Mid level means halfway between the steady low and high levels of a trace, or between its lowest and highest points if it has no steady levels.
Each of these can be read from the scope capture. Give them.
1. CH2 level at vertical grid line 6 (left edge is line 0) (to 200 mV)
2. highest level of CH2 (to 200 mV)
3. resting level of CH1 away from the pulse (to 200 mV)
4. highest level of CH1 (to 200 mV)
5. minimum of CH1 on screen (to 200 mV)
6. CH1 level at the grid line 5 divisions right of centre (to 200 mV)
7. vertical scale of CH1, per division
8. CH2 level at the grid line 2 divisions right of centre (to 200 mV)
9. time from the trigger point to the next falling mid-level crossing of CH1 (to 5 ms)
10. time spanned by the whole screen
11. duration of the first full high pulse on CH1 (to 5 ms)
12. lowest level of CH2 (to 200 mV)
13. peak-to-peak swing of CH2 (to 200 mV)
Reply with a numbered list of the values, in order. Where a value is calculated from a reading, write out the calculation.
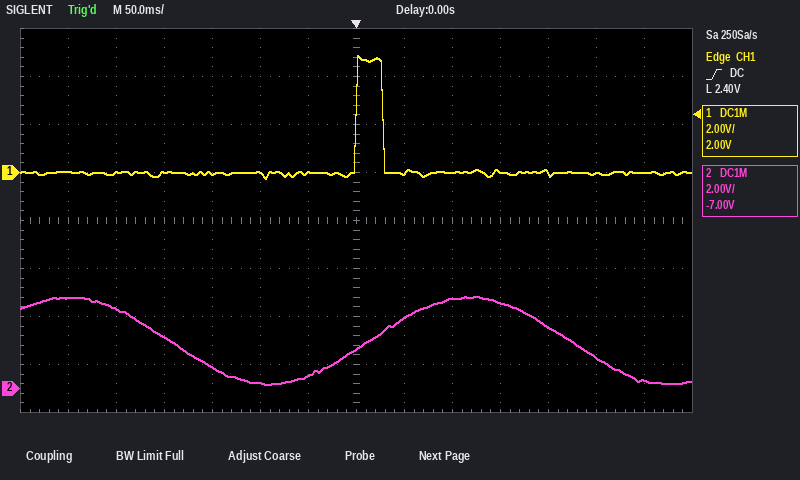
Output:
1. 600 mV
2. 3.8 V
3. 0.0 V
4. 4.8 V
5. -200 mV
6. 0.0 V
7. 2 V
8. 3.8 V
9. 30 ms
10. 700 ms
11. 30 ms
12. 200 mV
13. 3.8 V − (200 mV) = 3.6 V
